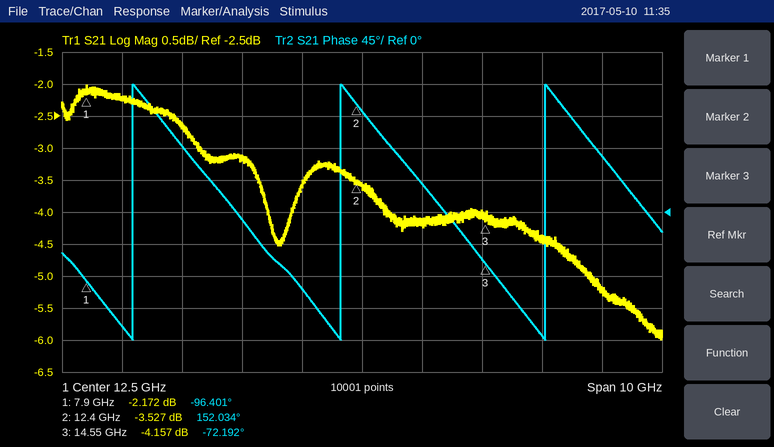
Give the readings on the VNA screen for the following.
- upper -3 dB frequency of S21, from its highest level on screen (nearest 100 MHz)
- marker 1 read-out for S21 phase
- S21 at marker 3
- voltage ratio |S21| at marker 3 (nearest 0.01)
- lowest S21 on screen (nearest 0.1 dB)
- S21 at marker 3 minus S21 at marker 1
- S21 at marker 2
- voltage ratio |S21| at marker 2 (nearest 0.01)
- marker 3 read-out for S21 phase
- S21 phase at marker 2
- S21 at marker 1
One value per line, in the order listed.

16.3 GHz
-96.401°
-4.157 dB
0.62
-6.0 dB
-1.985 dB
-3.527 dB
0.67
-72.192°
152.034°
-2.172 dB
